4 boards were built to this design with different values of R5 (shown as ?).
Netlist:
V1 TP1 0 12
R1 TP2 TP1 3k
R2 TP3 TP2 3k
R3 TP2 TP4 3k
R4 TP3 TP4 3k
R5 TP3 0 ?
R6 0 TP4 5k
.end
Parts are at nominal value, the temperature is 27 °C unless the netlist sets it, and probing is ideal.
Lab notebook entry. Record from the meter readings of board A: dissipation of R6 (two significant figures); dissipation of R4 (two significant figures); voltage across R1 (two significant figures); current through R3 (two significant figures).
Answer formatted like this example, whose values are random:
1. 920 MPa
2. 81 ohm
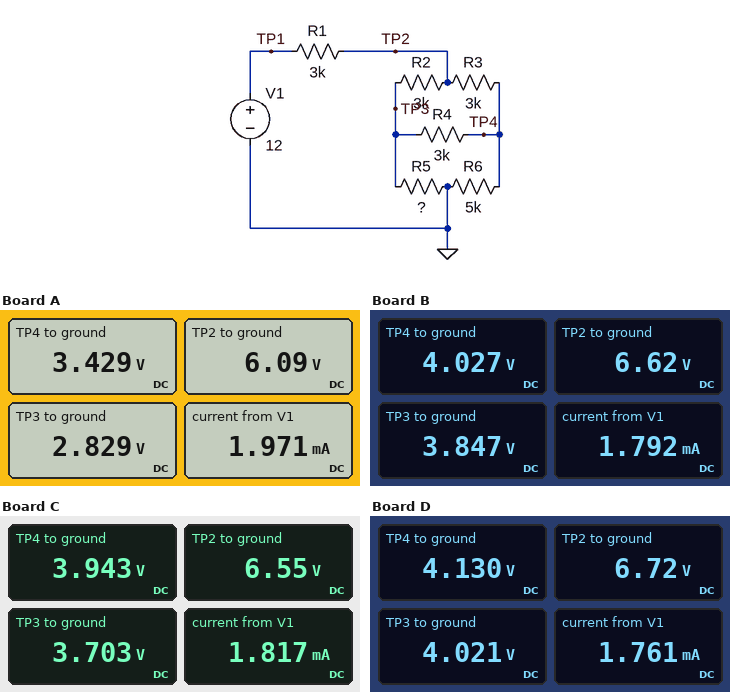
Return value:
1. 2.4 mW
2. 120 µW
3. 5.9 V
4. 890 µA
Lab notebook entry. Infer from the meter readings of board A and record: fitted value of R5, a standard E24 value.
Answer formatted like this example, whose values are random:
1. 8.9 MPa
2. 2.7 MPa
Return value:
1. 2.2 kΩ
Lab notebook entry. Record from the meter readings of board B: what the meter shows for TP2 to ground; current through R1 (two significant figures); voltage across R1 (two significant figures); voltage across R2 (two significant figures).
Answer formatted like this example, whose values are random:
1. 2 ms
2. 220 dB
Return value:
1. 6.62 V
2. 1.8 mA
3. 5.4 V
4. 2.8 V
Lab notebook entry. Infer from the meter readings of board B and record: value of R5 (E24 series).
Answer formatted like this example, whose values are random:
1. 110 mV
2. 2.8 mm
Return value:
1. 3.9 kΩ
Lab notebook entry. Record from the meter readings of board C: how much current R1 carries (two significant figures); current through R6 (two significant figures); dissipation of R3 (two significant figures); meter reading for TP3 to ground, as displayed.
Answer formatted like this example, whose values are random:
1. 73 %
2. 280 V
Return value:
1. 1.8 mA
2. 790 µA
3. 2.3 mW
4. 3.703 V
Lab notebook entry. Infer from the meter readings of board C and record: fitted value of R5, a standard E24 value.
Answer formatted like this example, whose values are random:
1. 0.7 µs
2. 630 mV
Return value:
1. 3.6 kΩ
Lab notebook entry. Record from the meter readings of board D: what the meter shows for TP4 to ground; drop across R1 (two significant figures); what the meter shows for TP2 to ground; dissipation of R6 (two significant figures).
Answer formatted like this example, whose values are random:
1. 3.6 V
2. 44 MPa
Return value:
1. 4.130 V
2. 5.3 V
3. 6.72 V
4. 3.4 mW
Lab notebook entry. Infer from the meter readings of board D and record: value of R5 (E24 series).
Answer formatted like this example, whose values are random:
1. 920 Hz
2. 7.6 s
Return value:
1. 4.3 kΩ
